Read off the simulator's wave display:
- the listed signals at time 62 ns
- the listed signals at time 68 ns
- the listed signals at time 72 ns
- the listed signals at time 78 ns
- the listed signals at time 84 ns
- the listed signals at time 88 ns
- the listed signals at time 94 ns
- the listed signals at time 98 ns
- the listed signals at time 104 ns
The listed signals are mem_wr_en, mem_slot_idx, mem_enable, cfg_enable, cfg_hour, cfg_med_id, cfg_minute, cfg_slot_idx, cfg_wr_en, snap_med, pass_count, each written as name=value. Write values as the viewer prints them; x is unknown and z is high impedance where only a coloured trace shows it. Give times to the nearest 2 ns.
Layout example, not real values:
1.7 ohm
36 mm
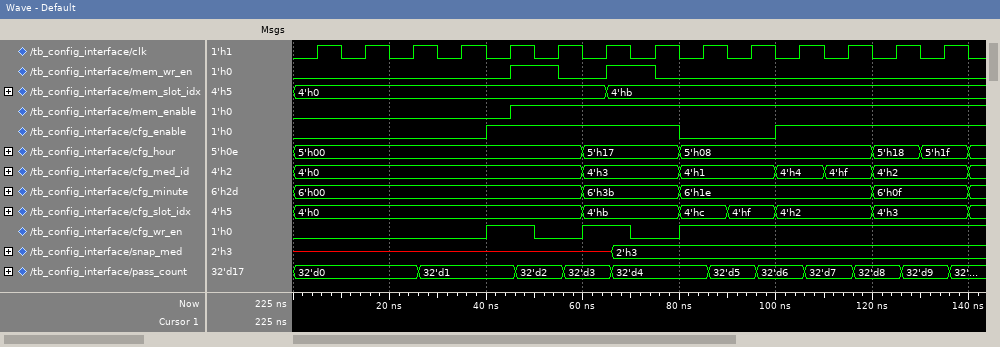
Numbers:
mem_wr_en=0, mem_slot_idx=4'h0, mem_enable=1, cfg_enable=1, cfg_hour=5'h17, cfg_med_id=4'h3, cfg_minute=6'h3b, cfg_slot_idx=4'hb, cfg_wr_en=1, snap_med=x, pass_count=32'd3
mem_wr_en=1, mem_slot_idx=4'hb, mem_enable=1, cfg_enable=1, cfg_hour=5'h17, cfg_med_id=4'h3, cfg_minute=6'h3b, cfg_slot_idx=4'hb, cfg_wr_en=1, snap_med=2'h3, pass_count=32'd4
mem_wr_en=1, mem_slot_idx=4'hb, mem_enable=1, cfg_enable=1, cfg_hour=5'h17, cfg_med_id=4'h3, cfg_minute=6'h3b, cfg_slot_idx=4'hb, cfg_wr_en=0, snap_med=2'h3, pass_count=32'd4
mem_wr_en=0, mem_slot_idx=4'hb, mem_enable=1, cfg_enable=1, cfg_hour=5'h17, cfg_med_id=4'h3, cfg_minute=6'h3b, cfg_slot_idx=4'hb, cfg_wr_en=0, snap_med=2'h3, pass_count=32'd4
mem_wr_en=0, mem_slot_idx=4'hb, mem_enable=1, cfg_enable=0, cfg_hour=5'h08, cfg_med_id=4'h1, cfg_minute=6'h1e, cfg_slot_idx=4'hc, cfg_wr_en=1, snap_med=2'h3, pass_count=32'd4
mem_wr_en=0, mem_slot_idx=4'hb, mem_enable=1, cfg_enable=0, cfg_hour=5'h08, cfg_med_id=4'h1, cfg_minute=6'h1e, cfg_slot_idx=4'hc, cfg_wr_en=1, snap_med=2'h3, pass_count=32'd5
mem_wr_en=0, mem_slot_idx=4'hb, mem_enable=1, cfg_enable=0, cfg_hour=5'h08, cfg_med_id=4'h1, cfg_minute=6'h1e, cfg_slot_idx=4'hf, cfg_wr_en=1, snap_med=2'h3, pass_count=32'd5
mem_wr_en=0, mem_slot_idx=4'hb, mem_enable=1, cfg_enable=0, cfg_hour=5'h08, cfg_med_id=4'h1, cfg_minute=6'h1e, cfg_slot_idx=4'hf, cfg_wr_en=1, snap_med=2'h3, pass_count=32'd6
mem_wr_en=0, mem_slot_idx=4'hb, mem_enable=1, cfg_enable=1, cfg_hour=5'h08, cfg_med_id=4'h4, cfg_minute=6'h1e, cfg_slot_idx=4'h2, cfg_wr_en=1, snap_med=2'h3, pass_count=32'd6
